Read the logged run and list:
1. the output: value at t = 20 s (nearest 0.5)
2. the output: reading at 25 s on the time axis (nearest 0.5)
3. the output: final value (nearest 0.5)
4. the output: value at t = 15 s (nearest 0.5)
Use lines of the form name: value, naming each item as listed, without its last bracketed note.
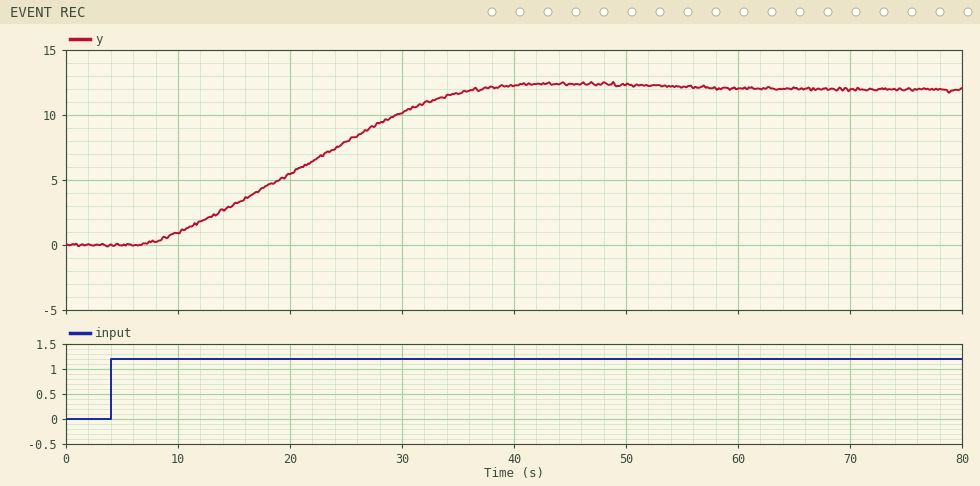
the output: value at t = 20 s: 5.5
the output: reading at 25 s on the time axis: 8.0
the output: final value: 12.0
the output: value at t = 15 s: 3.0
